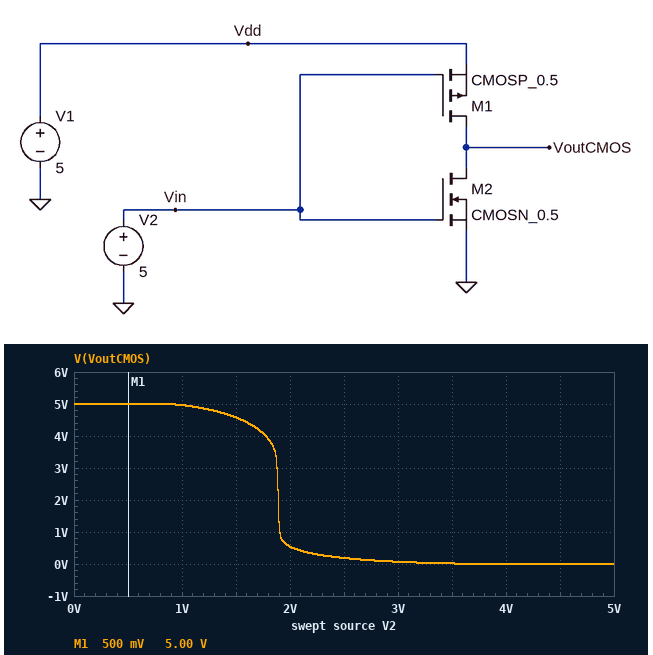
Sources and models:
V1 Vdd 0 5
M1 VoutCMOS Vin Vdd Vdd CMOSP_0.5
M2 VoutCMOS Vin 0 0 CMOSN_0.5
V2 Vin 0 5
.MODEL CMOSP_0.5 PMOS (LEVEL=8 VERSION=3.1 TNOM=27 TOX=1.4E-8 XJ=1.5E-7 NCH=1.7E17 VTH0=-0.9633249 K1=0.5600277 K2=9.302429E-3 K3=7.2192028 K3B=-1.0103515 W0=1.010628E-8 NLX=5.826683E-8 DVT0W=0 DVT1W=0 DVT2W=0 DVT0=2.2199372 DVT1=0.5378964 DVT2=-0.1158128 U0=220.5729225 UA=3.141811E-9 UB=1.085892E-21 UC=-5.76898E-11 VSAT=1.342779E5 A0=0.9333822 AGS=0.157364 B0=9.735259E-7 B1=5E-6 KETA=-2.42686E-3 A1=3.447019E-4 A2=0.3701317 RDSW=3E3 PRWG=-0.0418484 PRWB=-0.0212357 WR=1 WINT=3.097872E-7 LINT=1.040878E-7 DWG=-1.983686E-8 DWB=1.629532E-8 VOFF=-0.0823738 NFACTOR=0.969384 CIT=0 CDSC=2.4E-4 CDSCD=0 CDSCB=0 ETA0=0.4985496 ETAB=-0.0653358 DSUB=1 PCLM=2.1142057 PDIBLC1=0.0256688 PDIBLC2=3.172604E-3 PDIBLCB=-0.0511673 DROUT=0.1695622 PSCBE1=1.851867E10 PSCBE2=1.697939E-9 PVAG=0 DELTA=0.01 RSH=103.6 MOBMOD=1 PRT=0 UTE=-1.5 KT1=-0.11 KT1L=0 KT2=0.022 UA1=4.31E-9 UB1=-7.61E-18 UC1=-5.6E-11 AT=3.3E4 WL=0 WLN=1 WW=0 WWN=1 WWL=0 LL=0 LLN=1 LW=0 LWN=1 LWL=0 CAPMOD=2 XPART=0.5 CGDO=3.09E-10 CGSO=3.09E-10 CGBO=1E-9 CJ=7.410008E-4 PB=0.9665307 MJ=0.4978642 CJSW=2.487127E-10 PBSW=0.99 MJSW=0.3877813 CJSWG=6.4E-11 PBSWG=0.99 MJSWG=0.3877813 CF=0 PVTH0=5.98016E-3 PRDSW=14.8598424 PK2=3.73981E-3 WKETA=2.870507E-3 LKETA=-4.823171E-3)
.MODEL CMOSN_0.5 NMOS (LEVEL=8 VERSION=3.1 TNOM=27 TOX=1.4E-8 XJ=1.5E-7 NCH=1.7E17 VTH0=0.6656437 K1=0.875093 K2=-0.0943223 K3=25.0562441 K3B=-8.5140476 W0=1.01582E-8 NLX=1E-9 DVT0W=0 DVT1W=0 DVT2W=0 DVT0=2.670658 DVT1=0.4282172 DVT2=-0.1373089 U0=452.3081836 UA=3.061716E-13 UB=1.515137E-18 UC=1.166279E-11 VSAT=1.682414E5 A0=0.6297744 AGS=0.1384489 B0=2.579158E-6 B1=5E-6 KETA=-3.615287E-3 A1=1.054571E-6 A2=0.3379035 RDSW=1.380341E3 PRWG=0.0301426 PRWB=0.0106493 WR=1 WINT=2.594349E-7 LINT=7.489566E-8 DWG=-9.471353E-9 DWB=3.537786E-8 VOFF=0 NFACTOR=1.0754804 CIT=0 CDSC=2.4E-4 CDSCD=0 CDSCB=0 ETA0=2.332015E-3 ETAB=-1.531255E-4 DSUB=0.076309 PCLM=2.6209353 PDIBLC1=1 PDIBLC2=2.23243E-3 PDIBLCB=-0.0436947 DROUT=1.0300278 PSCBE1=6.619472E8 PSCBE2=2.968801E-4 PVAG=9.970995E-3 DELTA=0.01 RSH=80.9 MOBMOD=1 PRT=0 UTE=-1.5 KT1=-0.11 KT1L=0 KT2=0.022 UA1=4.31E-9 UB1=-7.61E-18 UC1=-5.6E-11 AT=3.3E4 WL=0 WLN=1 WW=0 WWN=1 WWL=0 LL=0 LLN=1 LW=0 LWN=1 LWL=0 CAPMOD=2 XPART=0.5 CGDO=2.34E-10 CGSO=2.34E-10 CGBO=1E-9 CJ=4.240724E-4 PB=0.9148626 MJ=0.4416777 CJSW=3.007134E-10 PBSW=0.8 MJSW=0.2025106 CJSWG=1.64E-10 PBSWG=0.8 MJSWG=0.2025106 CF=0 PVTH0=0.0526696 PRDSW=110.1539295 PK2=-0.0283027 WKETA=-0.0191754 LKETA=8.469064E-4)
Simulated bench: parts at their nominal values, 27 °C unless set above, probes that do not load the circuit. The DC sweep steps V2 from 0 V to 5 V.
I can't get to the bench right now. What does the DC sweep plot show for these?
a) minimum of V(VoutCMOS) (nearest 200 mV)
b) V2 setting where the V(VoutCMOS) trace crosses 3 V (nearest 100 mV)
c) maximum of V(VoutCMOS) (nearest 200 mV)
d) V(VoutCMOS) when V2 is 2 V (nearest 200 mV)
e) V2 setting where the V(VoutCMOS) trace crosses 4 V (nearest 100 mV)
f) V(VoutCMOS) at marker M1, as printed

0 V
1.9 V
5.0 V
600 mV
1.8 V
5.00 V
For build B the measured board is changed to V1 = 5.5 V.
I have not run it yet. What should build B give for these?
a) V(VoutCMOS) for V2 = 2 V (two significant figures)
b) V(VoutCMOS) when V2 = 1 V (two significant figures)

4.0 V
5.5 V
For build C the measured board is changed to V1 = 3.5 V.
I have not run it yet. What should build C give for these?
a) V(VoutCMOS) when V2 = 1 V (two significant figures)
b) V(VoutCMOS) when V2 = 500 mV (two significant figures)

3.4 V
3.5 V
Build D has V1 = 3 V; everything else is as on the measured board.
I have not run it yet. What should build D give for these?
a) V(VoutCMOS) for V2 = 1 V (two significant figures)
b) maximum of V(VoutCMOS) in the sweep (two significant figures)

2.9 V
3.0 V
